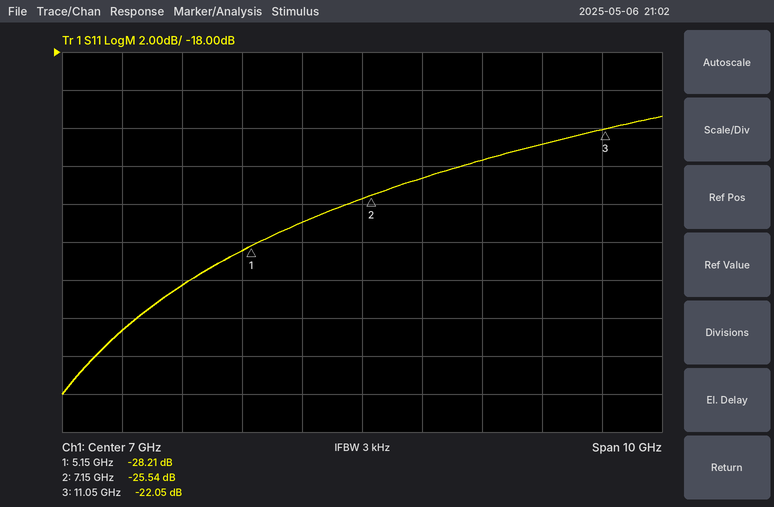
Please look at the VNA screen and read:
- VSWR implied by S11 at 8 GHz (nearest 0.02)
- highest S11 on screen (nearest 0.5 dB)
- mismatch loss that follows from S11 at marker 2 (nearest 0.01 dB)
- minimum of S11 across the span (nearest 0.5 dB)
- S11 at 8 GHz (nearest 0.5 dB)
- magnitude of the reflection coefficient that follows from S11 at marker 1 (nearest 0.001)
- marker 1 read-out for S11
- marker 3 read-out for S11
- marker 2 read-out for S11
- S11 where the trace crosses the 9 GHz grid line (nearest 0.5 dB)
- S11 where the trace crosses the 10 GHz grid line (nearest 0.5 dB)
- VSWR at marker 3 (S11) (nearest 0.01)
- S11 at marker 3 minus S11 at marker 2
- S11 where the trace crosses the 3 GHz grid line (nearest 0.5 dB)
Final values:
1.12
-21.5 dB
0.01 dB
-36.0 dB
-24.5 dB
0.039
-28.21 dB
-22.05 dB
-25.54 dB
-23.5 dB
-23.0 dB
1.17
3.49 dB
-32.5 dB
